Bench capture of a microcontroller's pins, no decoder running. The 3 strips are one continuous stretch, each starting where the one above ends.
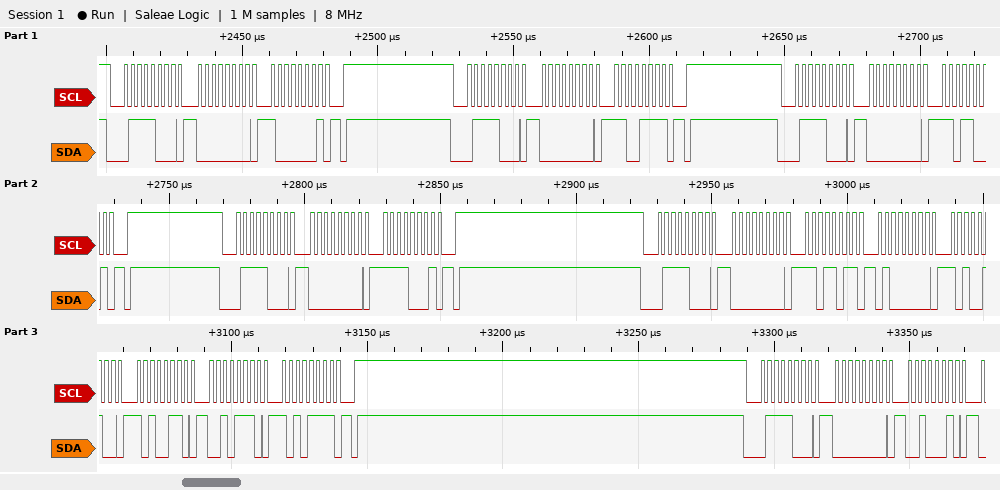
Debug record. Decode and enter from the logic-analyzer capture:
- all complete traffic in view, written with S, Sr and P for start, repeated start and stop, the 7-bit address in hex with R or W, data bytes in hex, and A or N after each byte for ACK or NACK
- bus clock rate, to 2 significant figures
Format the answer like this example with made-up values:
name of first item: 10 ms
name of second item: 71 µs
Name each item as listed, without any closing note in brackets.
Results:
all complete traffic in view, written with S, Sr and P for start, repeated start and stop, the 7-bit address in hex with R or W, data bytes in hex, and A or N after each byte for ACK or NACK: S 3CW A 00 A 81 A P S 3CW A 00 A CF A P S 3CW A 00 A D9 A P S 3CW A 00 A F1 A P S 3CW A 00 A DB A 40 A A4 A A6 A 2E A AF A P S 3CW A 00 A 22 A
bus clock rate, to 2 significant figures: 400 kHz
